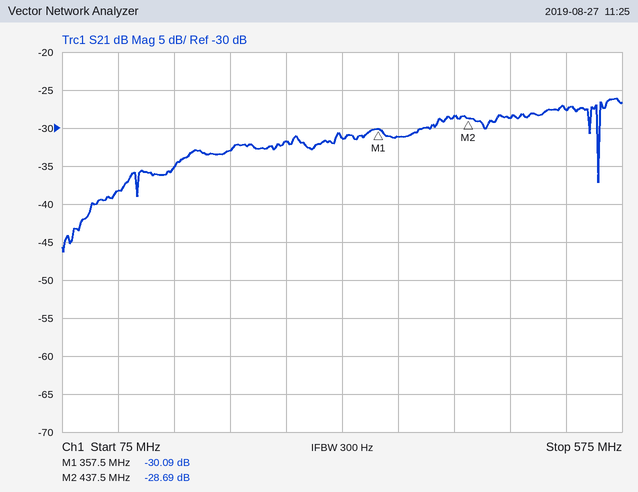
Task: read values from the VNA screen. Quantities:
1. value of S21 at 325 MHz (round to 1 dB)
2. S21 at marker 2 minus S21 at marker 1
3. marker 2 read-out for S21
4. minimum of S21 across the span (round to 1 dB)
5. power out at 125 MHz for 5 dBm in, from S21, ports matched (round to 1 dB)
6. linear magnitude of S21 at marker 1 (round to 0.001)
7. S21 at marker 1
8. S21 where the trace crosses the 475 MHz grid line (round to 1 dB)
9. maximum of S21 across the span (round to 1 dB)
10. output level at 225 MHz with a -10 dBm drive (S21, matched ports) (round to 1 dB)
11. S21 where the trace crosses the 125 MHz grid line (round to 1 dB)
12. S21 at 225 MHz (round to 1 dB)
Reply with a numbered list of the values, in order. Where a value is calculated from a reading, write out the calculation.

1. -31 dB
2. -28.69 − (-30.09) = 1.40 dB
3. -28.69 dB
4. -46 dB
5. 5 dBm + (-38 dB) = -33 dBm
6. 10^(-30.09/20) ≈ 0.031
7. -30.09 dB
8. -29 dB
9. -26 dB
10. -10 dBm + (-33 dB) = -43 dBm
11. -38 dB
12. -33 dB
